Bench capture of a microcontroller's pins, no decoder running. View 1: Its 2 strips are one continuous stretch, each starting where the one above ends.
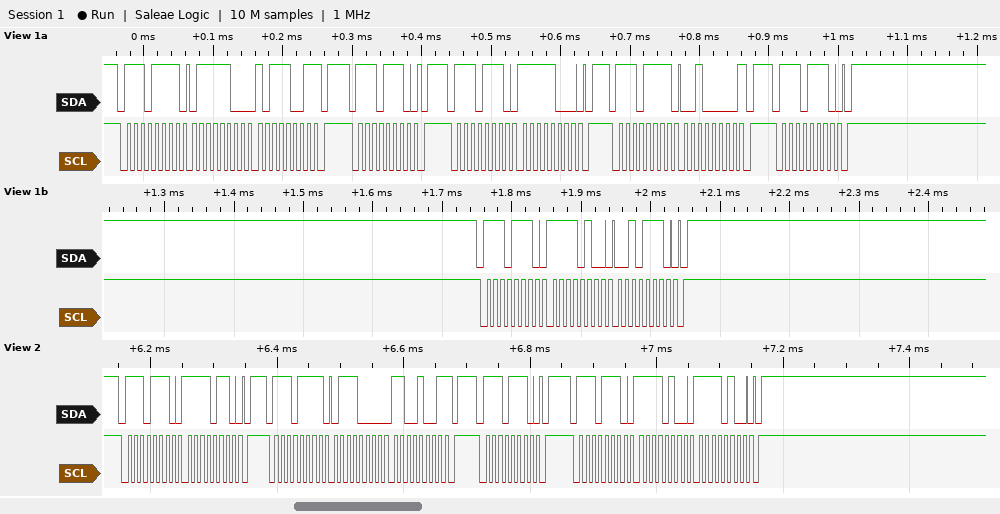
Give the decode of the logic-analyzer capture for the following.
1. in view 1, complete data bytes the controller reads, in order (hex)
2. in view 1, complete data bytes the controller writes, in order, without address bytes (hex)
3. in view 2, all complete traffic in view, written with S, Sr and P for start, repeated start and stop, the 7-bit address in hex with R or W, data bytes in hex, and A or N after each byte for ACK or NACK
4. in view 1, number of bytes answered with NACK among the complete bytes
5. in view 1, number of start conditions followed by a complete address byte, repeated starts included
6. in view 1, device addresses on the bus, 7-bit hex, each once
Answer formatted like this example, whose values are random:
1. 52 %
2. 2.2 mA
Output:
1. 7C B9 20
2. F8 F4 2E
3. S 77W A F6 A P S 77R A 70 A C9 N P S 77W A P S 77W A F4 A F4 A P
4. 2
5. 6
6. 0x77
